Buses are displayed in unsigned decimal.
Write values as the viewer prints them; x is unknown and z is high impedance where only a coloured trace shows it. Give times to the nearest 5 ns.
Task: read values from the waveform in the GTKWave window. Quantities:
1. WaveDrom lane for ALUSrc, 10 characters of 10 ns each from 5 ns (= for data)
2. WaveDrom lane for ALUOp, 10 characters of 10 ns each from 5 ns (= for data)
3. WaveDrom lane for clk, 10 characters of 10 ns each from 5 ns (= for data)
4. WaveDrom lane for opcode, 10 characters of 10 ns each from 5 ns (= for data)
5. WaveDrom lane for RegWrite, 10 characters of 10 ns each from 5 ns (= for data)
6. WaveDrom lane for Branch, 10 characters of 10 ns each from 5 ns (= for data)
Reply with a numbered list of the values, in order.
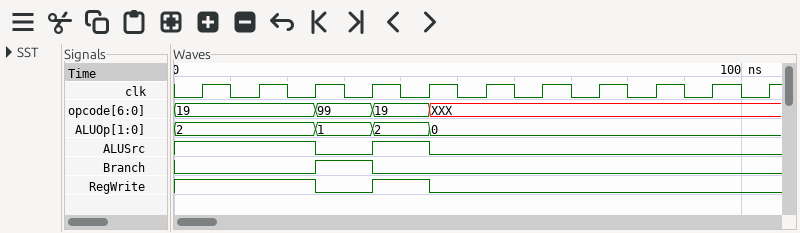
1. {name: 'ALUSrc', wave: '1.010.....'}
2. {name: 'ALUOp', wave: '=.===.....', data: '2 1 2 0'}
3. {name: 'clk', wave: 'p.........'}
4. {name: 'opcode', wave: '=.==x.....', data: '19 99 19'}
5. {name: 'RegWrite', wave: '1.010.....'}
6. {name: 'Branch', wave: '0.10......'}
